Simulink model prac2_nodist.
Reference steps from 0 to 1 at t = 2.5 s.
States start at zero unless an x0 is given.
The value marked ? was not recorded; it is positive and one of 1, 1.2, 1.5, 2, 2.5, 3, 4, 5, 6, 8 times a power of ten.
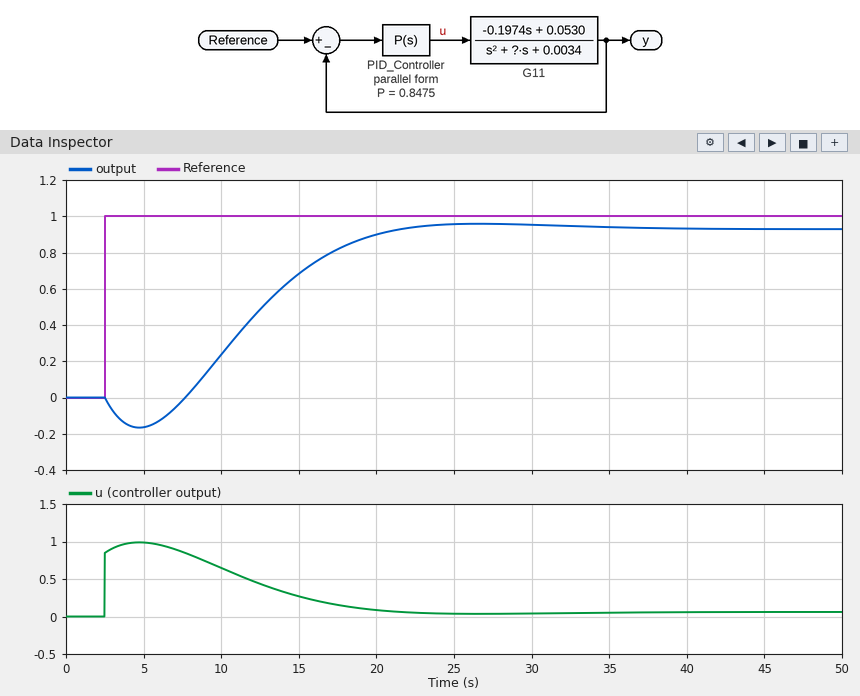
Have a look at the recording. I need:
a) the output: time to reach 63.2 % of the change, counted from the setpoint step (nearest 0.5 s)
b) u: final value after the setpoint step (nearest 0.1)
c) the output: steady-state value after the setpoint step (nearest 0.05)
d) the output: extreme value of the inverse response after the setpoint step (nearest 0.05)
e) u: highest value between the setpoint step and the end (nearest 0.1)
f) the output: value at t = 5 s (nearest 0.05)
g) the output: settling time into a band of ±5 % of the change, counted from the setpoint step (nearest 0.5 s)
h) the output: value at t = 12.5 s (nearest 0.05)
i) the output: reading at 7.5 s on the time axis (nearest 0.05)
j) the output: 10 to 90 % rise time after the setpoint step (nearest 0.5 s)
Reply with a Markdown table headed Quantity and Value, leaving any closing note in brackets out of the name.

| Quantity | Value |
|---|---|
| the output: time to reach 63.2 % of the change, counted from the setpoint step | 11.0 s |
| u: final value after the setpoint step | 0.1 |
| the output: steady-state value after the setpoint step | 0.95 |
| the output: extreme value of the inverse response after the setpoint step | -0.15 |
| u: highest value between the setpoint step and the end | 1.0 |
| the output: value at t = 5 s | -0.15 |
| the output: settling time into a band of ±5 % of the change, counted from the setpoint step | 17.0 s |
| the output: value at t = 12.5 s | 0.50 |
| the output: reading at 7.5 s on the time axis | 0.00 |
| the output: 10 to 90 % rise time after the setpoint step | 9.5 s |
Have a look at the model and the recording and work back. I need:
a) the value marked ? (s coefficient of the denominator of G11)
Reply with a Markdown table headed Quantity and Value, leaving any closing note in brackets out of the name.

| Quantity | Value |
|---|---|
| the value marked ? | 0.5 |
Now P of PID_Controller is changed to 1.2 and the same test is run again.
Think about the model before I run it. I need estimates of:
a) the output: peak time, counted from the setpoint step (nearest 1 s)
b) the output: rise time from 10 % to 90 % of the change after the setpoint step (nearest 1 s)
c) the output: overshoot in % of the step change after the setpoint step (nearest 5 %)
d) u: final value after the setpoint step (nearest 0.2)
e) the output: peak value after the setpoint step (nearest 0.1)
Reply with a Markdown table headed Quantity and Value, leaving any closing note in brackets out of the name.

| Quantity | Value |
|---|---|
| the output: peak time, counted from the setpoint step | 16 s |
| the output: rise time from 10 % to 90 % of the change after the setpoint step | 5 s |
| the output: overshoot in % of the step change after the setpoint step | 20 % |
| u: final value after the setpoint step | 0.0 |
| the output: peak value after the setpoint step | 1.1 |
